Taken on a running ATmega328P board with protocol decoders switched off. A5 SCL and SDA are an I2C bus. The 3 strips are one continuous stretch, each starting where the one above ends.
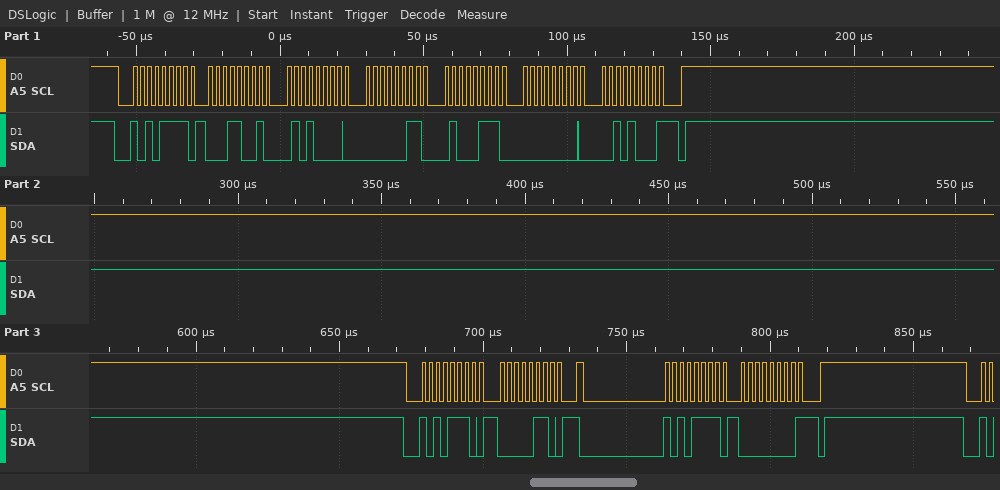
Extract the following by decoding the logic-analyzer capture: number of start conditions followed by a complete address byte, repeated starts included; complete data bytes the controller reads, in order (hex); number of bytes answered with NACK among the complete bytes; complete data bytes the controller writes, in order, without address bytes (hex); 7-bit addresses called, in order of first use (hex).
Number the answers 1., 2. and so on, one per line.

1. 3
2. 19 50 03 47 00 28 00
3. 2
4. 06
5. 0x57
